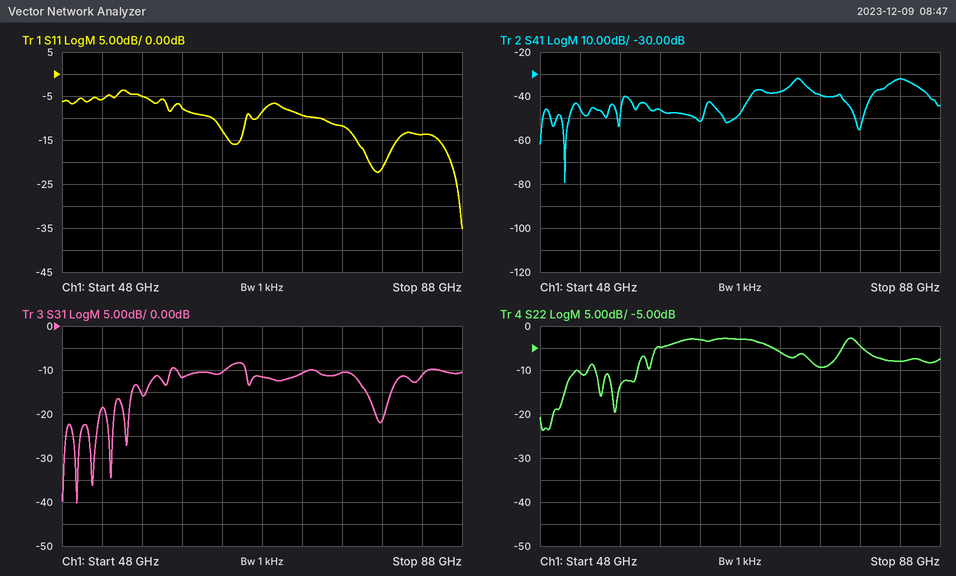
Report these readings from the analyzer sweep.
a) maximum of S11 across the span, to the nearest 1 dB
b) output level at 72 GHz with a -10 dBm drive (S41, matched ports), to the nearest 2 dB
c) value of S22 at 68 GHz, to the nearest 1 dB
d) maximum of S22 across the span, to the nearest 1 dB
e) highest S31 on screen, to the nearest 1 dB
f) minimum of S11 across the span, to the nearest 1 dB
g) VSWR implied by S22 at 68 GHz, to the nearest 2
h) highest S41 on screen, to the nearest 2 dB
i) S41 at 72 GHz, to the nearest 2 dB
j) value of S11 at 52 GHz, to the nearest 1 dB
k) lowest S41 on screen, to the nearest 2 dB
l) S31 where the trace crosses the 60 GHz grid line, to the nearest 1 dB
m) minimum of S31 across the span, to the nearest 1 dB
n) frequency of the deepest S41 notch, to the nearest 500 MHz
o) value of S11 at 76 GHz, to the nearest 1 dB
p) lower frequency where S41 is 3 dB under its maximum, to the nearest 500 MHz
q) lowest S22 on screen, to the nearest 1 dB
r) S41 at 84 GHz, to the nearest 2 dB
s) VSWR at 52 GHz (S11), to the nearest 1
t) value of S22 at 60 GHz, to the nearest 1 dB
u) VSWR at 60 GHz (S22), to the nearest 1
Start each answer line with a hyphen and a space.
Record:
- -4 dB
- -48 dBm
- -3 dB
- -3 dB
- -8 dB
- -35 dB
- 6
- -32 dB
- -38 dB
- -6 dB
- -80 dB
- -12 dB
- -40 dB
- 50.5 GHz
- -12 dB
- 73.0 GHz
- -24 dB
- -32 dB
- 3
- -5 dB
- 4
